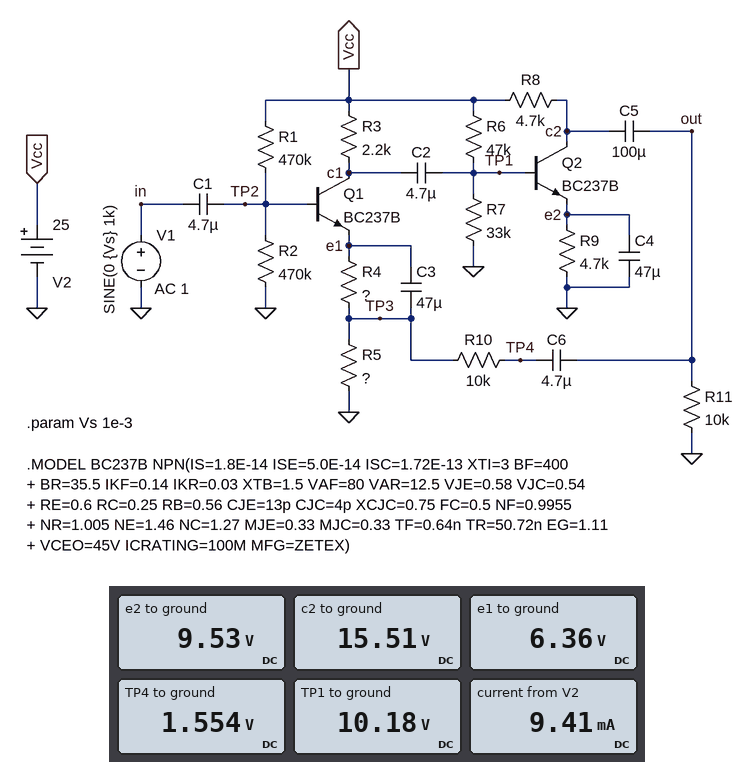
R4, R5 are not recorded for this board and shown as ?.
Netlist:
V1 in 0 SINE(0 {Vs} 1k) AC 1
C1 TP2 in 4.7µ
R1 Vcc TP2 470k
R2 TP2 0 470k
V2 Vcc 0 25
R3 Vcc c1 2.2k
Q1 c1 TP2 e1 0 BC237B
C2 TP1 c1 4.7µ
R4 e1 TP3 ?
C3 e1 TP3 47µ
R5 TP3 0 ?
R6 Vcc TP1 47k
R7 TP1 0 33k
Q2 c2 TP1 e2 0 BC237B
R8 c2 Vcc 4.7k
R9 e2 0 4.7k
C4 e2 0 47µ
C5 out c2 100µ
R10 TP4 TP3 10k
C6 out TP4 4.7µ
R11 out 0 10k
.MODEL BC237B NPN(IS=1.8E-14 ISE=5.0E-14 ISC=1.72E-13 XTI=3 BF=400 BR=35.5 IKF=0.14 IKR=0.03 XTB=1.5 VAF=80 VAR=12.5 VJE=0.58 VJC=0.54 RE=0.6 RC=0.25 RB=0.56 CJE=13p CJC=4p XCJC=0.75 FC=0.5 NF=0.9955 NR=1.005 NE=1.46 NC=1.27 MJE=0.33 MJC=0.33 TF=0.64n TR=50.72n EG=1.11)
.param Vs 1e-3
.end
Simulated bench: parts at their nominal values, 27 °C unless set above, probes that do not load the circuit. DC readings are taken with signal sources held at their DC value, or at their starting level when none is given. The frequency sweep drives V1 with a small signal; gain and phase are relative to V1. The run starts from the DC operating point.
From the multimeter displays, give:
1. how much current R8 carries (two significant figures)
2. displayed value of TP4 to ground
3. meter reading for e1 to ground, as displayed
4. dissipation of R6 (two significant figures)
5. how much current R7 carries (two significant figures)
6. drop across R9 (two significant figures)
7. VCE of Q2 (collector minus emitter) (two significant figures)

2.0 mA
1.554 V
6.36 V
4.7 mW
310 µA
9.5 V
6.0 V
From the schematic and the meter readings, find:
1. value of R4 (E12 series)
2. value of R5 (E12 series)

680 Ω
220 Ω
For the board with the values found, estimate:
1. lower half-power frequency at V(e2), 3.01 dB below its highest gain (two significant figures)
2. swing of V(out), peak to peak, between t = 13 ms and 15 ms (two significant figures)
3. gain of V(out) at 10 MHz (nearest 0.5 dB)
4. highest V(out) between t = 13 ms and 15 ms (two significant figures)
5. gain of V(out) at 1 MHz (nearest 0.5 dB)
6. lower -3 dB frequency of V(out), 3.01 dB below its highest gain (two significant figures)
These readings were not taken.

7.7 Hz
89 mV
28.5 dB
44 mV
33.0 dB
9.7 Hz
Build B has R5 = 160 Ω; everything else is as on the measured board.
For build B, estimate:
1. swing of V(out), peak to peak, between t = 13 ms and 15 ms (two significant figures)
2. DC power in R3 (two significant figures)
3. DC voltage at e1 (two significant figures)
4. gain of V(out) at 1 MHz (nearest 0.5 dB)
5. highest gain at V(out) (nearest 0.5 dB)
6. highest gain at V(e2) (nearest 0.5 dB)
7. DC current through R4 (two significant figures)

120 mV
120 mW
6.1 V
35.5 dB
40.0 dB
19.5 dB
7.3 mA
